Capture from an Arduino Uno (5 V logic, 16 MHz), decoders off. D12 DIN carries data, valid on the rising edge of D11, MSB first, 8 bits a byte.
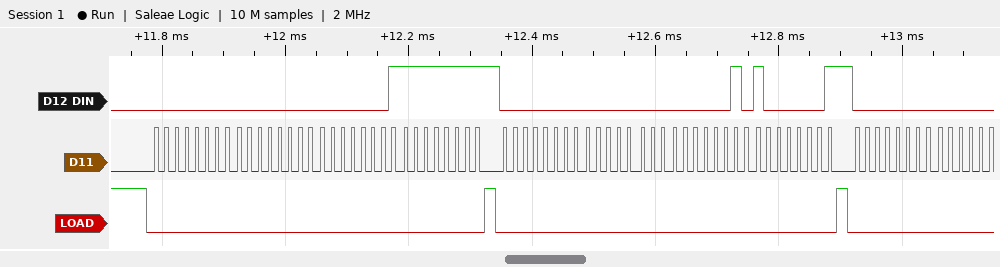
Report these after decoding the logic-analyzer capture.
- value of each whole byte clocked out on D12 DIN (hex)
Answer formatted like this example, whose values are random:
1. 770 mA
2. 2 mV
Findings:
1. 00 00 01 FF 00 00 02 81 00
